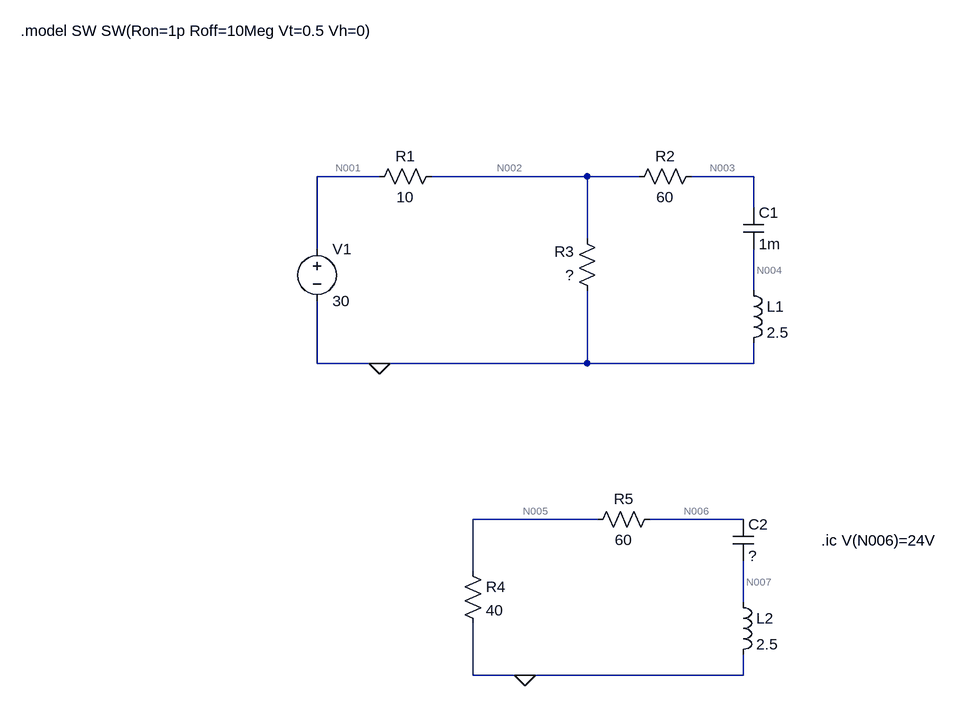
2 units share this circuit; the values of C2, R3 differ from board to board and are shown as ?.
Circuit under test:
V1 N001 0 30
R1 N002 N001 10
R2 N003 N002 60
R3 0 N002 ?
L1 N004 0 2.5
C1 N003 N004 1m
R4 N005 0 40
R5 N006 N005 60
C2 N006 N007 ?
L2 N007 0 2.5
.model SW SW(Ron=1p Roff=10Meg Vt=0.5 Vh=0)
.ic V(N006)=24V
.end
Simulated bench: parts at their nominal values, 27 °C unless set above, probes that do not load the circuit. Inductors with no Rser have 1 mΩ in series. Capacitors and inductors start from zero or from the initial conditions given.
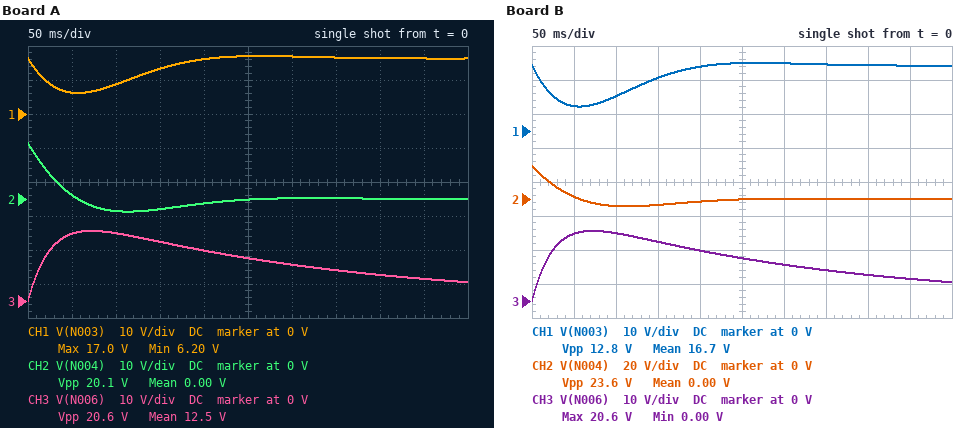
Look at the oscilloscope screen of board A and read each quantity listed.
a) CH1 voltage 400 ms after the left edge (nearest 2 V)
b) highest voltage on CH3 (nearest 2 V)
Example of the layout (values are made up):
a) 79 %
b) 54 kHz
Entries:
a) 16 V
b) 20 V
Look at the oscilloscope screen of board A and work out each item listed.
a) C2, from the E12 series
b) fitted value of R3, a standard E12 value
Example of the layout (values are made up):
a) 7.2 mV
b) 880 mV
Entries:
a) 3.3 mF
b) 12 Ω
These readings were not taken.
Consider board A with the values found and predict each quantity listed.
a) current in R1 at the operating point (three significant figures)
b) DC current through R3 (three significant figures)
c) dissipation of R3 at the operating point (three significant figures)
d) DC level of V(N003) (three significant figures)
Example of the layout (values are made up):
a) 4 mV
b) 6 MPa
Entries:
a) 1.36 A
b) 1.36 A
c) 22.3 W
d) 16.4 V
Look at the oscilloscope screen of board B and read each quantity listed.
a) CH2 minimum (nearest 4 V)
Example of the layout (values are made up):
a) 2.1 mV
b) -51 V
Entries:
a) -4 V
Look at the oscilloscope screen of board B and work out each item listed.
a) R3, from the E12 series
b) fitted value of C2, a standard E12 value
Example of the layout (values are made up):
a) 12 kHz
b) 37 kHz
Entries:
a) 18 Ω
b) 3.3 mF
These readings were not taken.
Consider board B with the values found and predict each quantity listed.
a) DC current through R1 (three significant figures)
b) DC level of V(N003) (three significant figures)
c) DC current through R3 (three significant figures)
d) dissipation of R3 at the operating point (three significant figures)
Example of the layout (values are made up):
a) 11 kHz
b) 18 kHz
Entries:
a) 1.07 A
b) 19.3 V
c) 1.07 A
d) 20.7 W
